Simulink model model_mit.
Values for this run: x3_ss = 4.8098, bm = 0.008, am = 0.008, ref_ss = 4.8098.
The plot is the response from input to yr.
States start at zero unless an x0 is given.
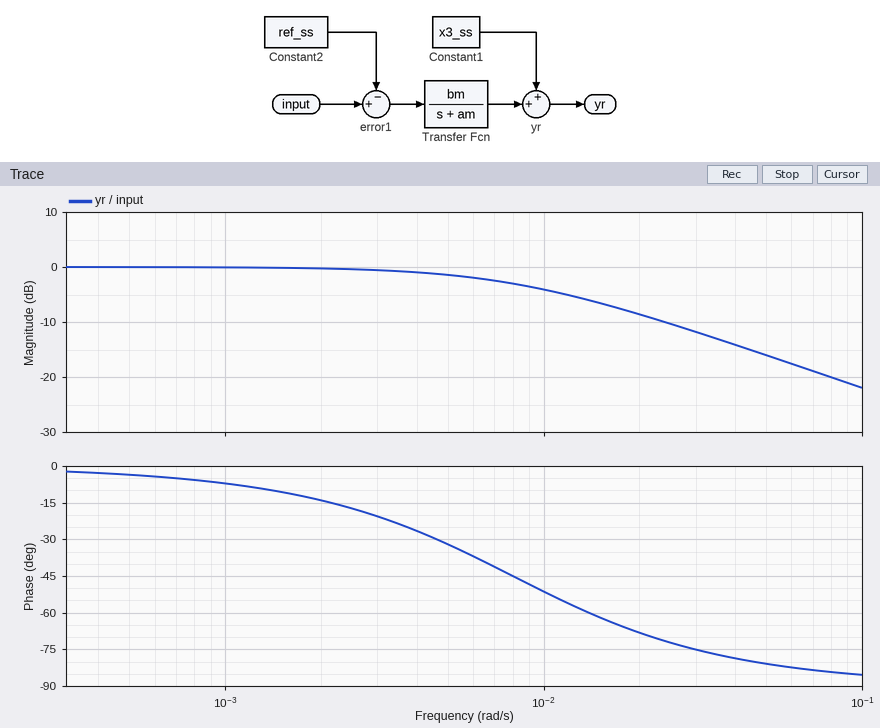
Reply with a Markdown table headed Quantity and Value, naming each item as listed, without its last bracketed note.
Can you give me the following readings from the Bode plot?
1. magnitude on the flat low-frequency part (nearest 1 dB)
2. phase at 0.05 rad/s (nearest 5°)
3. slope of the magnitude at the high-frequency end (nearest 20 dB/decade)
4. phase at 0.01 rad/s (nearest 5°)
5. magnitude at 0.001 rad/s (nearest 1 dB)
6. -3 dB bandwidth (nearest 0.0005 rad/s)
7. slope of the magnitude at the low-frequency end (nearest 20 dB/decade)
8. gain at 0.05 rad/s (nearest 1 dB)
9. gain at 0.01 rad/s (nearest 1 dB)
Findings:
| Quantity | Value |
|---|---|
| magnitude on the flat low-frequency part | 0 dB |
| phase at 0.05 rad/s | -80° |
| slope of the magnitude at the high-frequency end | -20 dB/decade |
| phase at 0.01 rad/s | -50° |
| magnitude at 0.001 rad/s | 0 dB |
| -3 dB bandwidth | 0.0080 rad/s |
| slope of the magnitude at the low-frequency end | 0 dB/decade |
| gain at 0.05 rad/s | -16 dB |
| gain at 0.01 rad/s | -4 dB |
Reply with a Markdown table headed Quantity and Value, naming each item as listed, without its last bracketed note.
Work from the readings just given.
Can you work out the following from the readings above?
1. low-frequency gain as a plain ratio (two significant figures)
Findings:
| Quantity | Value |
|---|---|
| low-frequency gain as a plain ratio | 1.0 |
